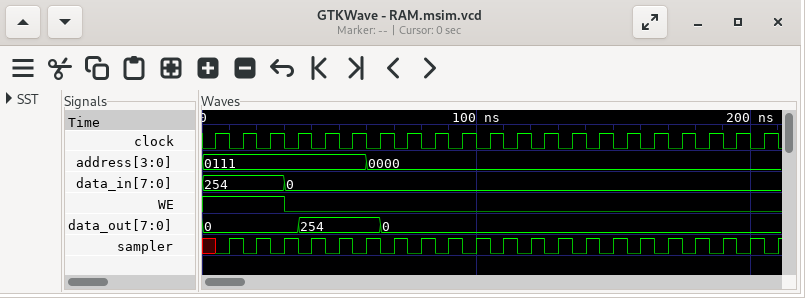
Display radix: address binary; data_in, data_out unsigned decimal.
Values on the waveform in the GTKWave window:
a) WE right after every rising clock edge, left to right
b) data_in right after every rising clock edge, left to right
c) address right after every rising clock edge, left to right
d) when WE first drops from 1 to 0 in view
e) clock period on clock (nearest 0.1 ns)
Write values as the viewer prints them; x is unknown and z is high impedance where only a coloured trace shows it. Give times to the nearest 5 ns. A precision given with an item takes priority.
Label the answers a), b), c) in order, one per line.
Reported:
a) 1 1 1 0 0 0 0 0 0 0 0 0 0 0 0 0 0 0 0 0 0
b) 254, 254, 254, 0, 0, 0, 0, 0, 0, 0, 0, 0, 0, 0, 0, 0, 0, 0, 0, 0, 0
c) 0111, 0111, 0111, 0111, 0111, 0111, 0000, 0000, 0000, 0000, 0000, 0000, 0000, 0000, 0000, 0000, 0000, 0000, 0000, 0000, 0000
d) 30 ns
e) 10 ns
